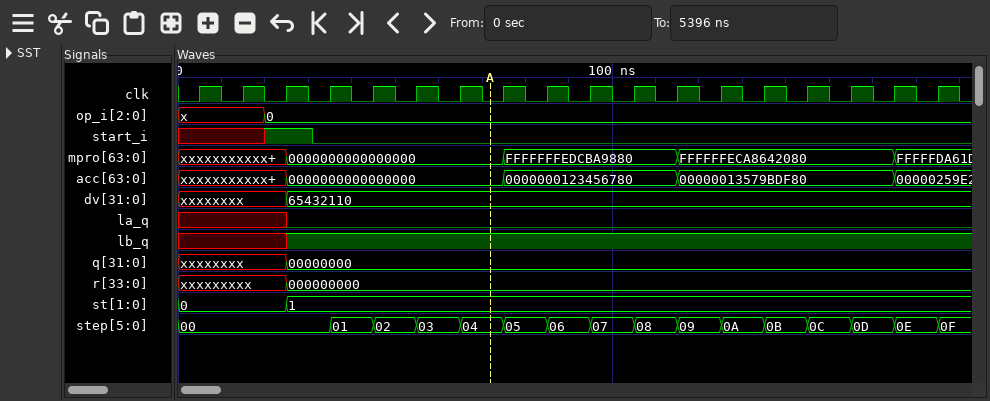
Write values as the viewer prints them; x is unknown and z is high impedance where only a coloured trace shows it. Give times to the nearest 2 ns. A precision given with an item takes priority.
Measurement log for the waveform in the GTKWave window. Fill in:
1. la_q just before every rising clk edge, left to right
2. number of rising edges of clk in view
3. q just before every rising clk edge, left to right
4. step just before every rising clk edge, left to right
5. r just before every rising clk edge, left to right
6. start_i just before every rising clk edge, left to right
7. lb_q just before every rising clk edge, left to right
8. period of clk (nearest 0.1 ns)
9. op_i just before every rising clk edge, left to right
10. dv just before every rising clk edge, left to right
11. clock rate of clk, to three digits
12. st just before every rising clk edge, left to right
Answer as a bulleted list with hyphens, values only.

- x x x 0 0 0 0 0 0 0 0 0 0 0 0 0 0 0
- 18
- xxxxxxxx, xxxxxxxx, xxxxxxxx, 00000000, 00000000, 00000000, 00000000, 00000000, 00000000, 00000000, 00000000, 00000000, 00000000, 00000000, 00000000, 00000000, 00000000, 00000000
- 00, 00, 00, 00, 01, 02, 03, 04, 05, 06, 07, 08, 09, 0A, 0B, 0C, 0D, 0E
- xxxxxxxxx, xxxxxxxxx, xxxxxxxxx, 000000000, 000000000, 000000000, 000000000, 000000000, 000000000, 000000000, 000000000, 000000000, 000000000, 000000000, 000000000, 000000000, 000000000, 000000000
- x x 1 0 0 0 0 0 0 0 0 0 0 0 0 0 0 0
- x x x 1 1 1 1 1 1 1 1 1 1 1 1 1 1 1
- 10 ns
- x, x, 0, 0, 0, 0, 0, 0, 0, 0, 0, 0, 0, 0, 0, 0, 0, 0
- xxxxxxxx, xxxxxxxx, xxxxxxxx, 65432110, 65432110, 65432110, 65432110, 65432110, 65432110, 65432110, 65432110, 65432110, 65432110, 65432110, 65432110, 65432110, 65432110, 65432110
- 100 MHz
- 0, 0, 0, 1, 1, 1, 1, 1, 1, 1, 1, 1, 1, 1, 1, 1, 1, 1
